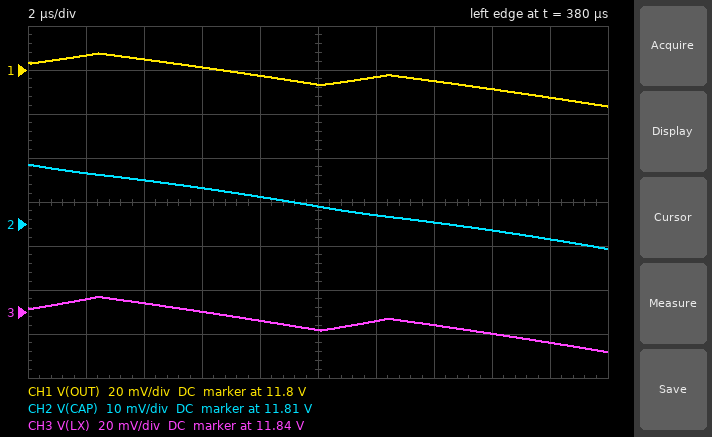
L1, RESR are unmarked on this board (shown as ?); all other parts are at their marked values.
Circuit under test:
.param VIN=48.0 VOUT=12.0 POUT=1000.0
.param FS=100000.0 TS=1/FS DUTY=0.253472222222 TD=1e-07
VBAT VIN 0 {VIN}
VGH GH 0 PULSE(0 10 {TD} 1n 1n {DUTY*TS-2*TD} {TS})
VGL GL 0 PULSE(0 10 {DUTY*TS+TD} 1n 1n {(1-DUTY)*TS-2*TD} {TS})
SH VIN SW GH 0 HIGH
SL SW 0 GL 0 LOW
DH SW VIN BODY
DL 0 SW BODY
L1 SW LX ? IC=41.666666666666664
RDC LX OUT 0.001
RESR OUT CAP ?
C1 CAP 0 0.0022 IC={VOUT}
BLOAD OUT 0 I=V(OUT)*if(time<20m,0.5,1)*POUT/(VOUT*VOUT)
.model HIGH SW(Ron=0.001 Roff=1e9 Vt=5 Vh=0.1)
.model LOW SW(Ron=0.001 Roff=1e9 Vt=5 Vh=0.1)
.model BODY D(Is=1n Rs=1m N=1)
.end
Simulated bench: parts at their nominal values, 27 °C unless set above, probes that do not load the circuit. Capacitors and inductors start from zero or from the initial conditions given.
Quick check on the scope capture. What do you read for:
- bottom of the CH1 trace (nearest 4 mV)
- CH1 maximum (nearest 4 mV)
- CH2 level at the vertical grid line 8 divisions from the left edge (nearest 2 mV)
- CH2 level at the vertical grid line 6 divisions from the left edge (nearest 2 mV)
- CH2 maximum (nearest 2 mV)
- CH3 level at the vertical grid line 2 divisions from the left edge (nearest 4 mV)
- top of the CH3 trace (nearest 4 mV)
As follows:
11.784 V
11.808 V
11.808 V
11.812 V
11.824 V
11.844 V
11.848 V
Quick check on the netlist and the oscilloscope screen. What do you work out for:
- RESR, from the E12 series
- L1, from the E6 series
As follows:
8.2 mΩ
100 µH
